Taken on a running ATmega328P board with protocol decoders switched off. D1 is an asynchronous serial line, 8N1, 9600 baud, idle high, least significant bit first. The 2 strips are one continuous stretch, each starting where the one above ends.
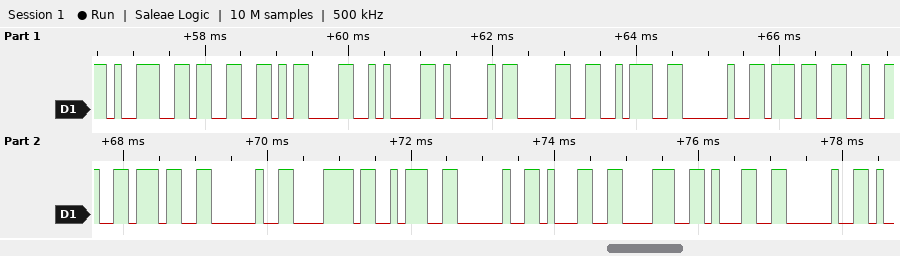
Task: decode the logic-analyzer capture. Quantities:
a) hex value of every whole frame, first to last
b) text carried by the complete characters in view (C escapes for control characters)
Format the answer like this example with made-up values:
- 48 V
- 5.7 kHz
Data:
- 0x39 0x33 0x0D 0x0A 0x41 0x30 0x3A 0x20 0x37 0x32 0x37 0x20 0x78 0x3A 0x20 0x31 0x38 0x31 0x20
- "93\r\nA0: 727 x: 181 "
